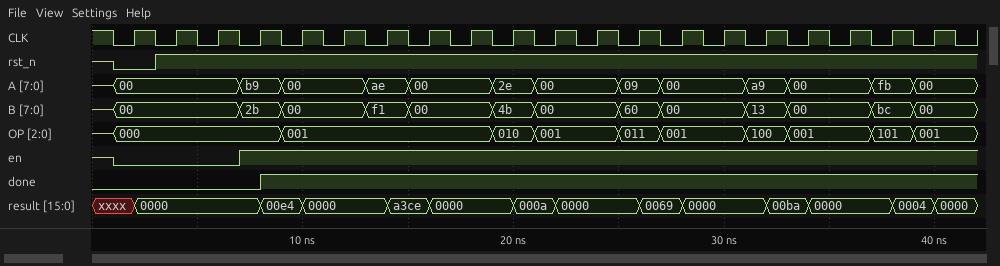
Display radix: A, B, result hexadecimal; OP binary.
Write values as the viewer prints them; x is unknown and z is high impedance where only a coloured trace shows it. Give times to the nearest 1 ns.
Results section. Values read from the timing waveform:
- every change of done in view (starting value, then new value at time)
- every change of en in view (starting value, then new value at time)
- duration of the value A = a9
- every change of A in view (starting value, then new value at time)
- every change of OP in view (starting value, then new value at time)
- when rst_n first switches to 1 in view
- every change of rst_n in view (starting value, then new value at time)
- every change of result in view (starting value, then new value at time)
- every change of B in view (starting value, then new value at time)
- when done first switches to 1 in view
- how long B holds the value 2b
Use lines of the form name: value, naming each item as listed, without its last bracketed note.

every change of done in view: 0, 1 at 8 ns
every change of en in view: z, 0 at 1 ns, 1 at 7 ns
duration of the value A = a9: 2 ns
every change of A in view: z, 00 at 1 ns, b9 at 7 ns, 00 at 9 ns, ae at 13 ns, 00 at 15 ns, 2e at 19 ns, 00 at 21 ns, 09 at 25 ns, 00 at 27 ns, a9 at 31 ns, 00 at 33 ns, fb at 37 ns, 00 at 39 ns
every change of OP in view: z, 000 at 1 ns, 001 at 9 ns, 010 at 19 ns, 001 at 21 ns, 011 at 25 ns, 001 at 27 ns, 100 at 31 ns, 001 at 33 ns, 101 at 37 ns, 001 at 39 ns
when rst_n first switches to 1 in view: 3 ns
every change of rst_n in view: z, 0 at 1 ns, 1 at 3 ns
every change of result in view: xxxx, 0000 at 2 ns, 00e4 at 8 ns, 0000 at 10 ns, a3ce at 14 ns, 0000 at 16 ns, 000a at 20 ns, 0000 at 22 ns, 0069 at 26 ns, 0000 at 28 ns, 00ba at 32 ns, 0000 at 34 ns, 0004 at 38 ns, 0000 at 40 ns
every change of B in view: z, 00 at 1 ns, 2b at 7 ns, 00 at 9 ns, f1 at 13 ns, 00 at 15 ns, 4b at 19 ns, 00 at 21 ns, 60 at 25 ns, 00 at 27 ns, 13 at 31 ns, 00 at 33 ns, bc at 37 ns, 00 at 39 ns
when done first switches to 1 in view: 8 ns
how long B holds the value 2b: 2 ns
